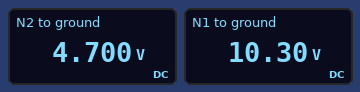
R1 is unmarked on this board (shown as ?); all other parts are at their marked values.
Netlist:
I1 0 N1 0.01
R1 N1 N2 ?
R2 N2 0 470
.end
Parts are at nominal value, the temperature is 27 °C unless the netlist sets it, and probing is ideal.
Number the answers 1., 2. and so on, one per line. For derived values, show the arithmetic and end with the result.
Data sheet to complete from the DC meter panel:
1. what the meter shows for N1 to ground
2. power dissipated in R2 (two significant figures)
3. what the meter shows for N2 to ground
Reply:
1. 10.30 V
2. (4.7 V)^2 / 470 Ω = 47 mW
3. 4.700 V
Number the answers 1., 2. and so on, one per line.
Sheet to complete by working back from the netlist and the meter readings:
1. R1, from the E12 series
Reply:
1. 560 Ω
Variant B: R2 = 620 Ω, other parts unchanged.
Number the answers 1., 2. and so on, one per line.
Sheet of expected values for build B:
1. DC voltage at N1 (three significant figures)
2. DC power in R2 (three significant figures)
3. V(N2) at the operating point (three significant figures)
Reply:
1. 11.8 V
2. 62.0 mW
3. 6.20 V
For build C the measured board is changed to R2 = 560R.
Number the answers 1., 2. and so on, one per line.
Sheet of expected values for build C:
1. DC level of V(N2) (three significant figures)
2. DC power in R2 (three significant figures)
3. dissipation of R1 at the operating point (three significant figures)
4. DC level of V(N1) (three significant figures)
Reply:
1. 5.60 V
2. 56.0 mW
3. 56.0 mW
4. 11.2 V
